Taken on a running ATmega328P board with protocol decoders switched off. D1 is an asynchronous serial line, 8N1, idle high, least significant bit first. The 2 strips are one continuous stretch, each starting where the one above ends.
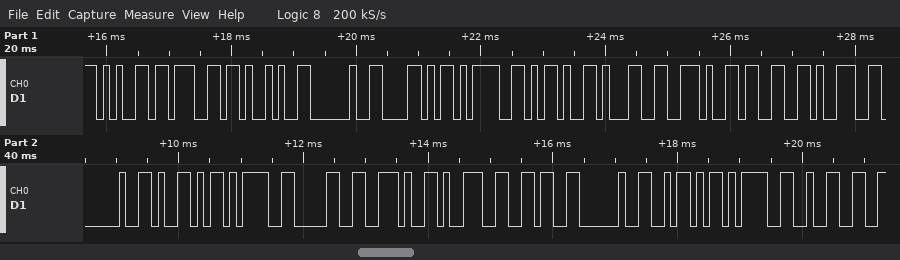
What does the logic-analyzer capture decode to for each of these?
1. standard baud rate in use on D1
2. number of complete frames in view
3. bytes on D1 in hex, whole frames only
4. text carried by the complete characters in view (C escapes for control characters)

9600 baud
22
65 67 29 20 58 3D 2D 31 2E 33 39 20 59 3D 30 2E 39 36 20 5A 3D 32
"eg) X=-1.39 Y=0.96 Z=2"
